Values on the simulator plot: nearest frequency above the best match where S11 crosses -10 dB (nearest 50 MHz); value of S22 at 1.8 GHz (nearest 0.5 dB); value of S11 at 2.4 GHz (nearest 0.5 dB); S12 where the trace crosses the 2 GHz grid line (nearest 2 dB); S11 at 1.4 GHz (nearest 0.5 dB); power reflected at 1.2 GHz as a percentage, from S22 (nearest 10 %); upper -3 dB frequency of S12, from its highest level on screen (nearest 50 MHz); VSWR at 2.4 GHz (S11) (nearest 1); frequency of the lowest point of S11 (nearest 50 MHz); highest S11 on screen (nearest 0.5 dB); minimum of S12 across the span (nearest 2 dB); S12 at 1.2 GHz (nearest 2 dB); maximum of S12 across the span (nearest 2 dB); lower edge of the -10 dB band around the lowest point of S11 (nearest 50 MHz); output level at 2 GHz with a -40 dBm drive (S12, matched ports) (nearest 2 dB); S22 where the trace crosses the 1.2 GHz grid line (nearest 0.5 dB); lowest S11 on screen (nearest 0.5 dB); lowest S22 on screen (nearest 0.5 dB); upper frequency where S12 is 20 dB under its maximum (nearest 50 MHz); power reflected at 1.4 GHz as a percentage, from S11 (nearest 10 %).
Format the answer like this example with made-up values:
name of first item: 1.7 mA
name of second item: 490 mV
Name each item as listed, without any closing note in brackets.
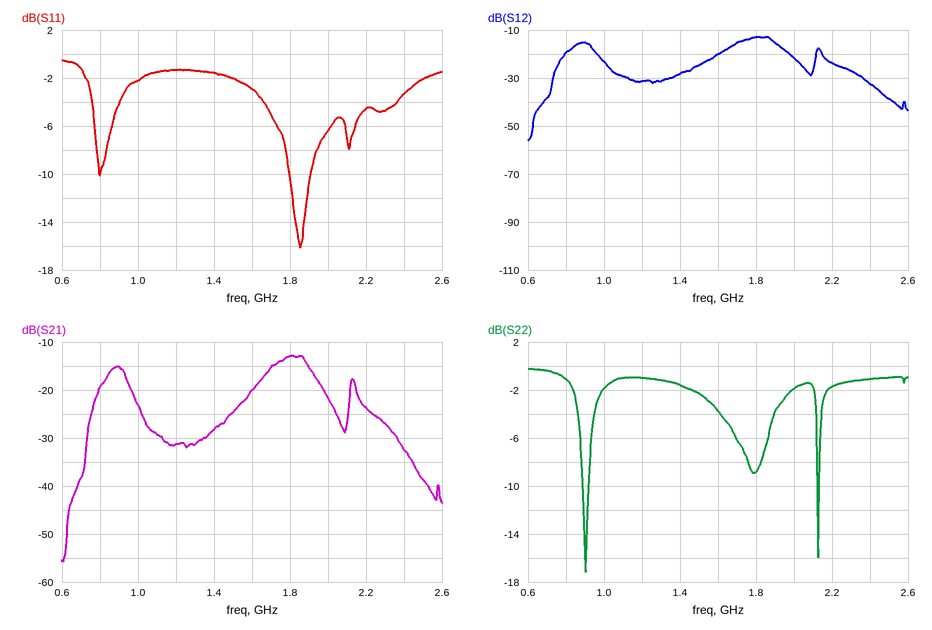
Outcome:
nearest frequency above the best match where S11 crosses -10 dB: 1.90 GHz
value of S22 at 1.8 GHz: -9.0 dB
value of S11 at 2.4 GHz: -3.5 dB
S12 where the trace crosses the 2 GHz grid line: -22 dB
S11 at 1.4 GHz: -1.5 dB
power reflected at 1.2 GHz as a percentage, from S22: 80 %
upper -3 dB frequency of S12, from its highest level on screen: 1.90 GHz
VSWR at 2.4 GHz (S11): 5
frequency of the lowest point of S11: 1.85 GHz
highest S11 on screen: -0.5 dB
minimum of S12 across the span: -56 dB
S12 at 1.2 GHz: -32 dB
maximum of S12 across the span: -12 dB
lower edge of the -10 dB band around the lowest point of S11: 1.80 GHz
output level at 2 GHz with a -40 dBm drive (S12, matched ports): -62 dBm
S22 where the trace crosses the 1.2 GHz grid line: -1.0 dB
lowest S11 on screen: -16.0 dB
lowest S22 on screen: -17.0 dB
upper frequency where S12 is 20 dB under its maximum: 2.40 GHz
power reflected at 1.4 GHz as a percentage, from S11: 70 %
